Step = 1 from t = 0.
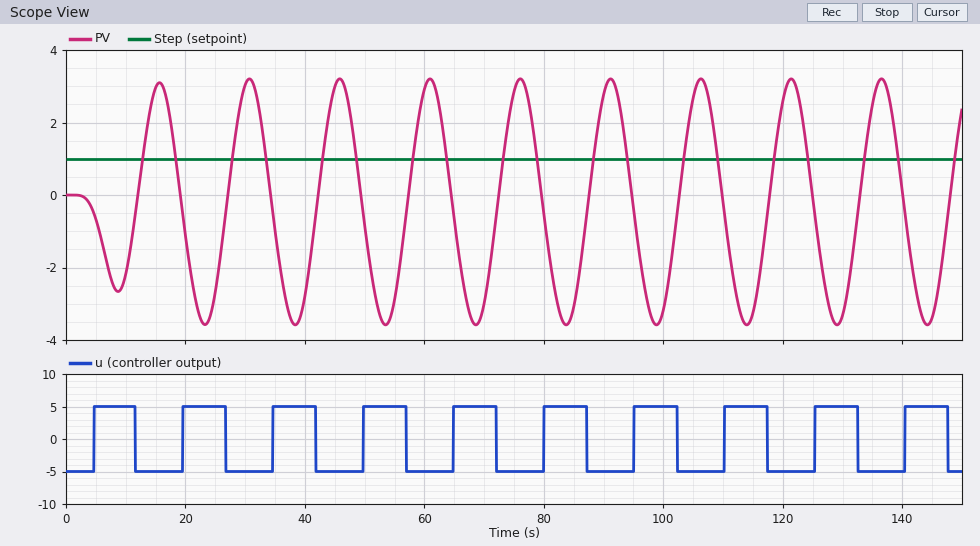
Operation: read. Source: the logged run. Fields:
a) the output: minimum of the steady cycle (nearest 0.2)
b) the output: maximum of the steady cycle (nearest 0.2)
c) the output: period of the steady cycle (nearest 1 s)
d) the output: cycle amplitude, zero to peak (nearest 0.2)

-3.6
3.2
15 s
3.4
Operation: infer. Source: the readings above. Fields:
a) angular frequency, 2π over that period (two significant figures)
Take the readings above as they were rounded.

0.42 rad/s
